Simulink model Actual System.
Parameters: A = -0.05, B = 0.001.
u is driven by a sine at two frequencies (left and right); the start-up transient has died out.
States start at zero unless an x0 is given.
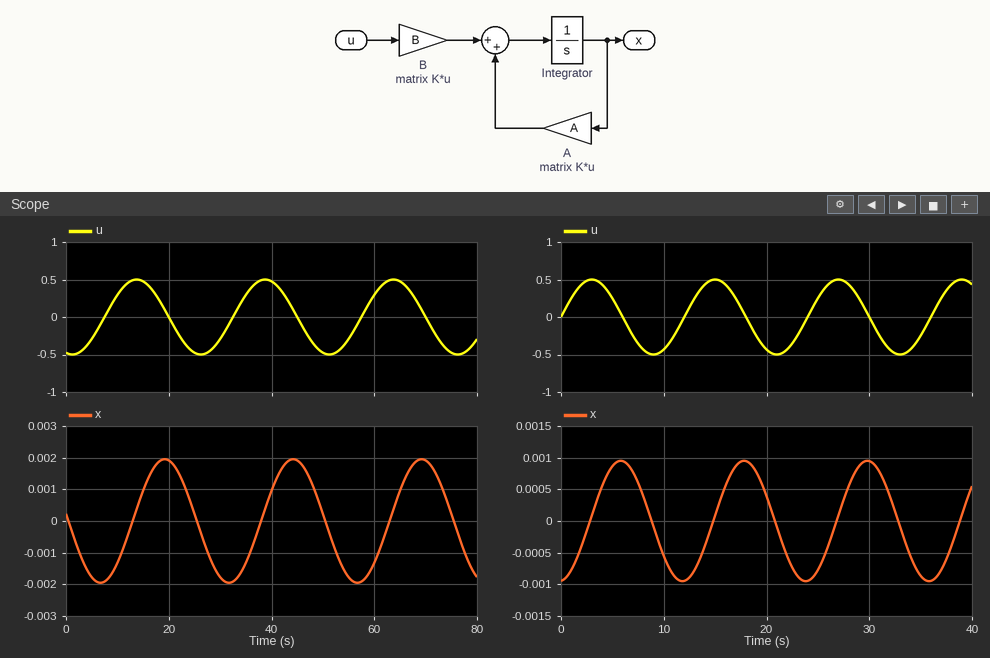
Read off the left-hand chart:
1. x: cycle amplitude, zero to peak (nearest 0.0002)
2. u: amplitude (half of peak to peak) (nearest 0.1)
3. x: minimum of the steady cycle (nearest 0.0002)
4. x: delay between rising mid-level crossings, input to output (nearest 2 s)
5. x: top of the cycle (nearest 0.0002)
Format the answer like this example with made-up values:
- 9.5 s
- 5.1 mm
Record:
- 0.0020
- 0.5
- -0.0020
- 6 s
- 0.0020
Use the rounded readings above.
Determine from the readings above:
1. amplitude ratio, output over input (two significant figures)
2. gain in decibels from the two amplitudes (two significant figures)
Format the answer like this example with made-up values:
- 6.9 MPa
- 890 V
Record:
- 0.0040
- -48 dB
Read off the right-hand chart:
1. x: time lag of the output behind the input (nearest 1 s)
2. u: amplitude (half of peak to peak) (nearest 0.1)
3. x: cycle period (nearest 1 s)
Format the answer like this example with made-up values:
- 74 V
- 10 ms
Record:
- 3 s
- 0.5
- 12 s
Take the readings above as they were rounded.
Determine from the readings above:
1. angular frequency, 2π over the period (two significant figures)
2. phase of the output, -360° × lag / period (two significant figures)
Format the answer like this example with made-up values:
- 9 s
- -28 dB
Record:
- 0.52 rad/s
- -90°
